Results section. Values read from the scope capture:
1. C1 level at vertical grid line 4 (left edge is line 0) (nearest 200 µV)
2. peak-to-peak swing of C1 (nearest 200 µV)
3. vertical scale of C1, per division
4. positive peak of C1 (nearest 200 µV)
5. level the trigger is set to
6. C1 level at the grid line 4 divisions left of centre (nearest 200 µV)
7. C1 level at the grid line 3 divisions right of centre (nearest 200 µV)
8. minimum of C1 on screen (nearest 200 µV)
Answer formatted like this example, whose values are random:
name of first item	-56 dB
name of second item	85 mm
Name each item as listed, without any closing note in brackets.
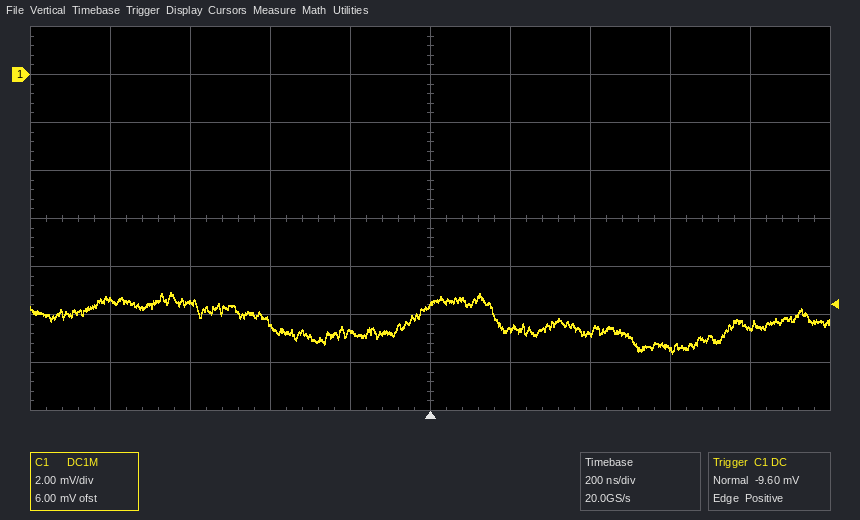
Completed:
C1 level at vertical grid line 4 (left edge is line 0)	-10.8 mV
peak-to-peak swing of C1	2.6 mV
vertical scale of C1, per division	2 mV
positive peak of C1	-9.0 mV
level the trigger is set to	-9.60 mV
C1 level at the grid line 4 divisions left of centre	-9.4 mV
C1 level at the grid line 3 divisions right of centre	-11.4 mV
minimum of C1 on screen	-11.6 mV
